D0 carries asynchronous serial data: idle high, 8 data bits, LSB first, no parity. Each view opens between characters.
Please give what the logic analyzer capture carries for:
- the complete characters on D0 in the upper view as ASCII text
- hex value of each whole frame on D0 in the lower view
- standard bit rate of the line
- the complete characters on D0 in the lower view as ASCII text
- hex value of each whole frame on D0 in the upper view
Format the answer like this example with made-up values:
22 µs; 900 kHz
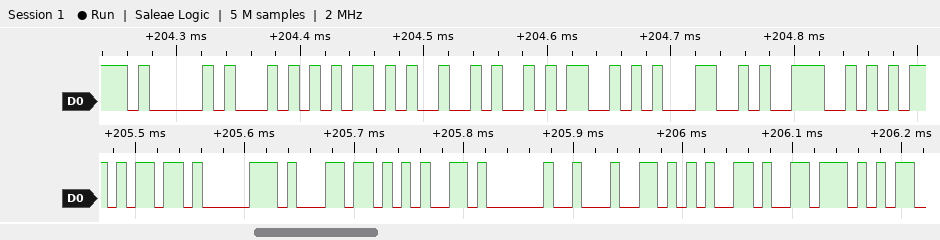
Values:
"AT+JSLN"; 6D, 70, 6C, 65, 20, 64, 65, 76; 115200 baud; "mple dev"; 41, 54, 2B, 4A, 53, 4C, 4E
